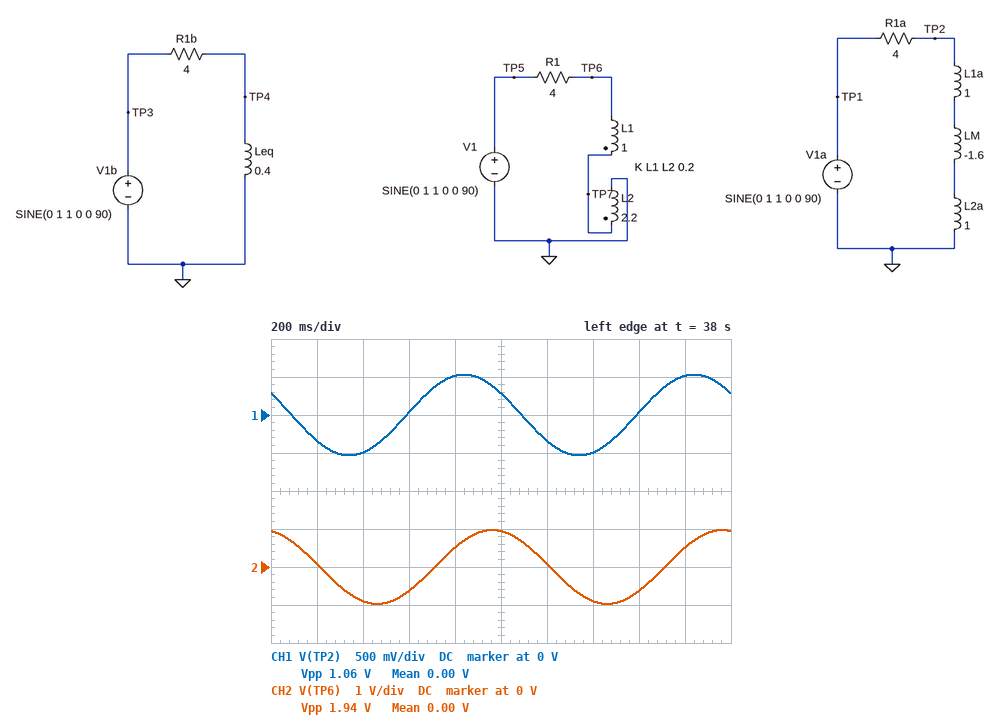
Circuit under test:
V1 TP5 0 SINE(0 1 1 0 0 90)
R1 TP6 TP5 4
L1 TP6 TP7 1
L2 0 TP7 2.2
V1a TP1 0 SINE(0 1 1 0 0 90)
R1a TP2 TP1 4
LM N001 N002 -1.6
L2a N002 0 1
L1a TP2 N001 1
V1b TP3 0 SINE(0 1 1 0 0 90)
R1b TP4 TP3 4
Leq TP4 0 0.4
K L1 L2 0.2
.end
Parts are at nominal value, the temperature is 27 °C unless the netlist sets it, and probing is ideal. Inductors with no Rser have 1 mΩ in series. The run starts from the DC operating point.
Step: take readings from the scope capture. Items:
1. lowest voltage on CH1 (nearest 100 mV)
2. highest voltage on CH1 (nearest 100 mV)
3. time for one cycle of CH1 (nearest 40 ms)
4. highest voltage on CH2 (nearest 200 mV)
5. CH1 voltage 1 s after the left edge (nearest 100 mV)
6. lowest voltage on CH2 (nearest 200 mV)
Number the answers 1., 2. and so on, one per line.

1. -500 mV
2. 500 mV
3. 1.00 s
4. 1.0 V
5. 300 mV
6. -1.0 V
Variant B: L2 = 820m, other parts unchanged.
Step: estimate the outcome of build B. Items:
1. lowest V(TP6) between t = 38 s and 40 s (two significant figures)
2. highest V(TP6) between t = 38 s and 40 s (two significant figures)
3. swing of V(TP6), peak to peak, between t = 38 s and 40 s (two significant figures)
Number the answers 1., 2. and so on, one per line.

1. -920 mV
2. 920 mV
3. 1.8 V
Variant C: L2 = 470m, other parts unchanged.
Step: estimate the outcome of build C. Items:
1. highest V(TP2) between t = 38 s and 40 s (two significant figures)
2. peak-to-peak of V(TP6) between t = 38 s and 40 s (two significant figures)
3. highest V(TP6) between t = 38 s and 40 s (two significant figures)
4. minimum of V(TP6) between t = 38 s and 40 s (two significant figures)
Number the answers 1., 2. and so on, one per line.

1. 530 mV
2. 1.8 V
3. 880 mV
4. -880 mV
